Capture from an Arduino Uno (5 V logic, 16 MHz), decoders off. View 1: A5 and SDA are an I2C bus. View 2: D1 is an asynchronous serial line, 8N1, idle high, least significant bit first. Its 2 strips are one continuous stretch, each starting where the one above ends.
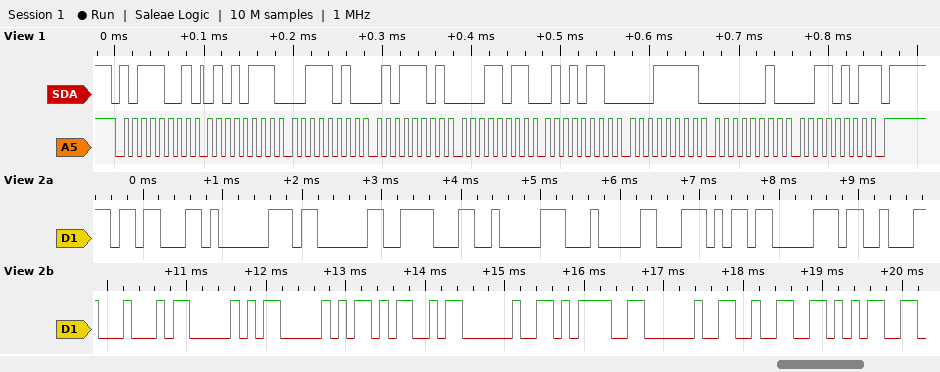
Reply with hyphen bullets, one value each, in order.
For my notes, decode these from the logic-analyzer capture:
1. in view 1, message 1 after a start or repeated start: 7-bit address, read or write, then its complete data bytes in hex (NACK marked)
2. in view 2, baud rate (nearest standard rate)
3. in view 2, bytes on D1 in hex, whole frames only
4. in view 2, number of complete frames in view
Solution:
- 0x5C read: 57 3A 5D 1B 56 1F 02 35 NACK
- 9600 baud
- 1B 81 03 1E 82 04 5C 83 13 44 50 50 4D 20 3D 20 32 35
- 18
